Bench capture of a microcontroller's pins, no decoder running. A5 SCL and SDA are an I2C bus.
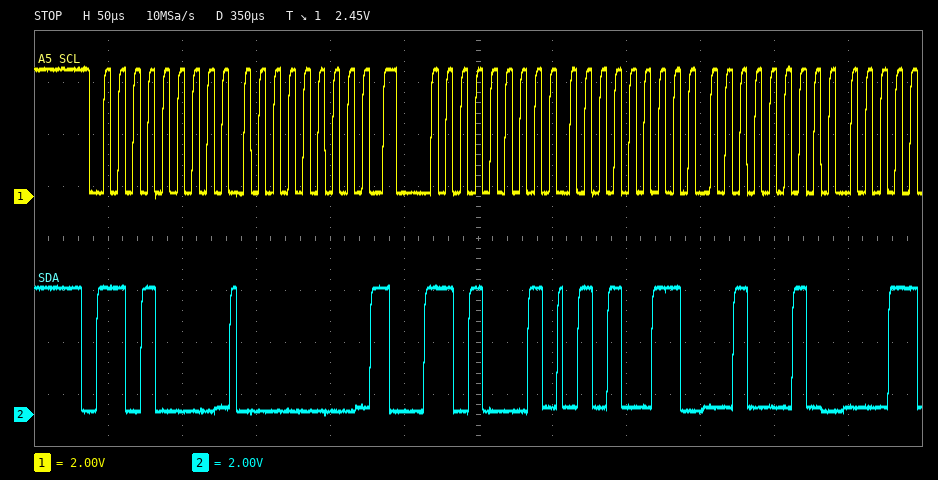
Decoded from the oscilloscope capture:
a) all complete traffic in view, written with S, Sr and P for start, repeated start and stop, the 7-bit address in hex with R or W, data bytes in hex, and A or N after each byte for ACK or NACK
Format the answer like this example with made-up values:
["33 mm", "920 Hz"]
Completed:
["S 68W A 00 A Sr 68R A 53 A 22 A"]
